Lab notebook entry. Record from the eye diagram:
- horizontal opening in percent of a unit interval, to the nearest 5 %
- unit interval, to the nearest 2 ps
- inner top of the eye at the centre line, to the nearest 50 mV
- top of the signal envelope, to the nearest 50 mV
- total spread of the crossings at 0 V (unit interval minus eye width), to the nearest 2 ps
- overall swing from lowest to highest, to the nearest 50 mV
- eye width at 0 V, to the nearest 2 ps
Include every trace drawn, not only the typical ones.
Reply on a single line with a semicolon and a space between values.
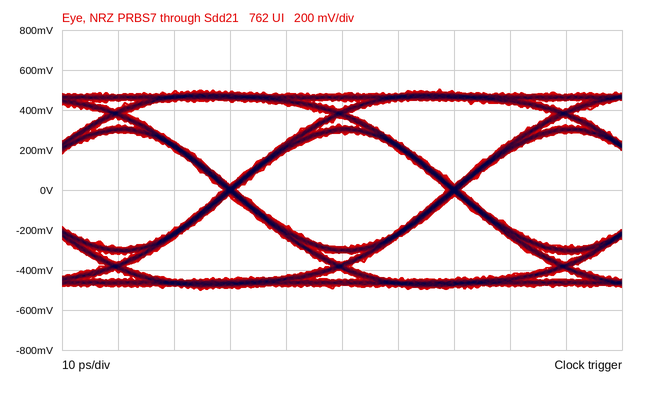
95 %; 40 ps; 300 mV; 500 mV; 2 ps; 1.00 V; 38 ps
